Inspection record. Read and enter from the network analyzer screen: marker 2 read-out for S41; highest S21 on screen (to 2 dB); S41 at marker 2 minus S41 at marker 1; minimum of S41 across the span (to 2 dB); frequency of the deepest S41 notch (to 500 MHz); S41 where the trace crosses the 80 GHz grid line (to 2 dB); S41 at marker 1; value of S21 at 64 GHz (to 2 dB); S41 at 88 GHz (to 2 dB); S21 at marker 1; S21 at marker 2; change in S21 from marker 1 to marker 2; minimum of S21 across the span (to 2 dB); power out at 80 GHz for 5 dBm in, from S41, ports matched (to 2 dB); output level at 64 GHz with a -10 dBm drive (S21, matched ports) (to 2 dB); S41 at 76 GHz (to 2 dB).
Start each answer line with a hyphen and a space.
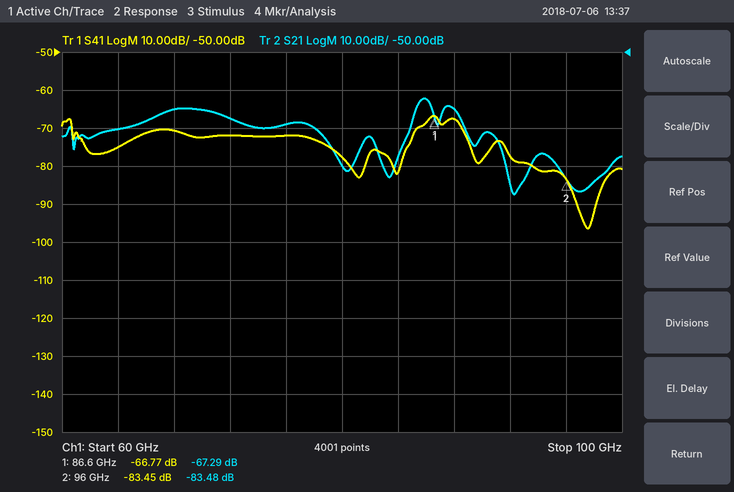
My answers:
- -83.45 dB
- -62 dB
- -16.68 dB
- -96 dB
- 97.5 GHz
- -78 dB
- -66.77 dB
- -70 dB
- -68 dB
- -67.29 dB
- -83.48 dB
- -16.19 dB
- -88 dB
- -72 dBm
- -80 dBm
- -72 dB
